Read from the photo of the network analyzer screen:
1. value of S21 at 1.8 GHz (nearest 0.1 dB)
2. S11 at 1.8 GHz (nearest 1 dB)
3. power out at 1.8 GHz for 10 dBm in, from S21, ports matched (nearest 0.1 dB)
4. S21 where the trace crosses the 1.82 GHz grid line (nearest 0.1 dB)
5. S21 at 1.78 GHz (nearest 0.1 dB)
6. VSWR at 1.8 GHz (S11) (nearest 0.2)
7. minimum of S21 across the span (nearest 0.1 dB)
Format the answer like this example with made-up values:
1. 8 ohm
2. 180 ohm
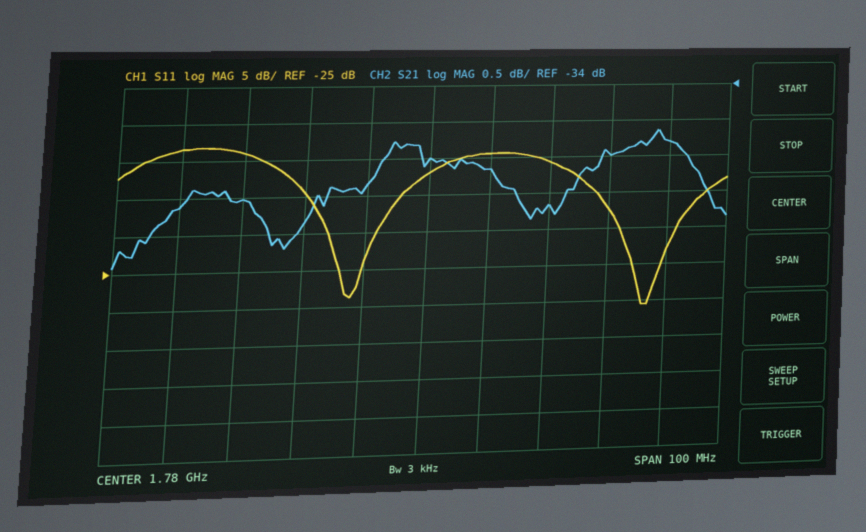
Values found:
1. -35.7 dB
2. -11 dB
3. -25.7 dBm
4. -34.8 dB
5. -35.0 dB
6. 1.8
7. -36.4 dB
